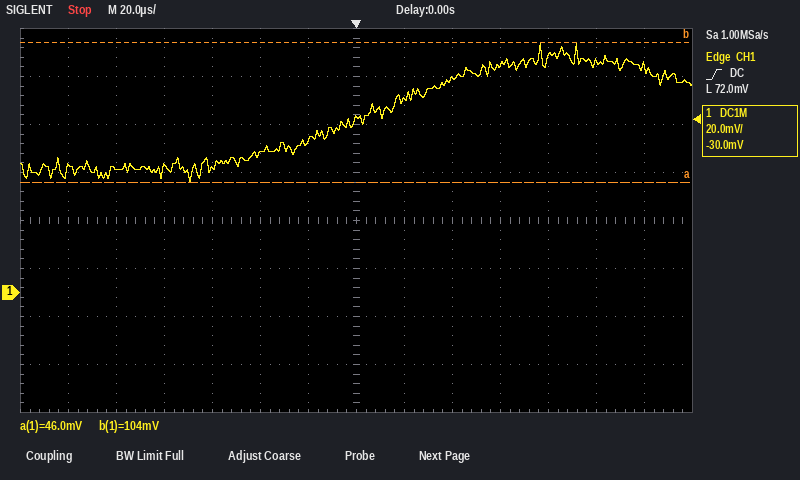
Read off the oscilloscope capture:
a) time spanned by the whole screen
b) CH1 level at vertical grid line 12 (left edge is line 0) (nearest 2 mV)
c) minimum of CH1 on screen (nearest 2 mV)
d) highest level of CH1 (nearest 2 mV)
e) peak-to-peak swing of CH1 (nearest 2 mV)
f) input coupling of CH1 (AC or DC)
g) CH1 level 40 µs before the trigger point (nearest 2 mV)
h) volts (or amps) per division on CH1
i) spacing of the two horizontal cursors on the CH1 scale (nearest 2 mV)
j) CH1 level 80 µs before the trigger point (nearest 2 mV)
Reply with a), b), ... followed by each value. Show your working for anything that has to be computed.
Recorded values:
a) 280 µs
b) 96 mV
c) 46 mV
d) 104 mV
e) 104 mV − (46 mV) = 58 mV
f) DC
g) 58 mV
h) 20 mV
i) 58 mV
j) 52 mV
